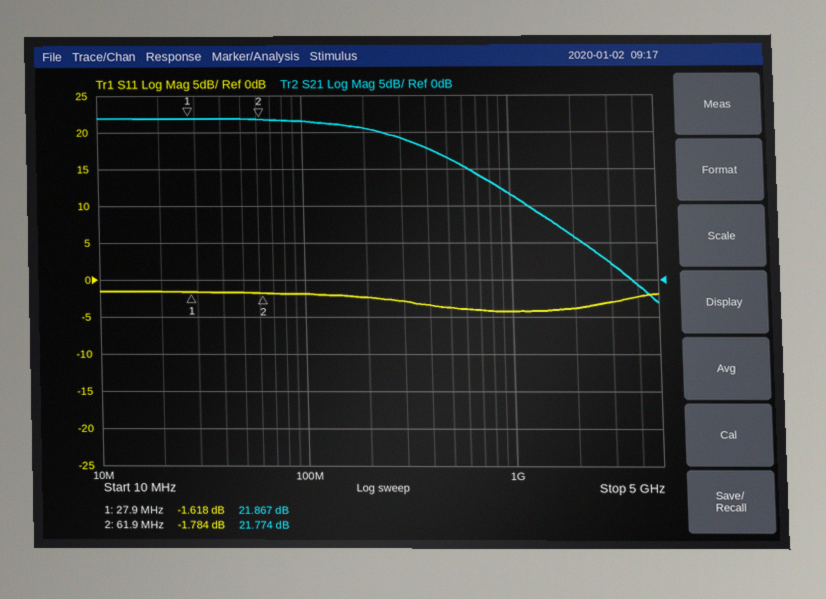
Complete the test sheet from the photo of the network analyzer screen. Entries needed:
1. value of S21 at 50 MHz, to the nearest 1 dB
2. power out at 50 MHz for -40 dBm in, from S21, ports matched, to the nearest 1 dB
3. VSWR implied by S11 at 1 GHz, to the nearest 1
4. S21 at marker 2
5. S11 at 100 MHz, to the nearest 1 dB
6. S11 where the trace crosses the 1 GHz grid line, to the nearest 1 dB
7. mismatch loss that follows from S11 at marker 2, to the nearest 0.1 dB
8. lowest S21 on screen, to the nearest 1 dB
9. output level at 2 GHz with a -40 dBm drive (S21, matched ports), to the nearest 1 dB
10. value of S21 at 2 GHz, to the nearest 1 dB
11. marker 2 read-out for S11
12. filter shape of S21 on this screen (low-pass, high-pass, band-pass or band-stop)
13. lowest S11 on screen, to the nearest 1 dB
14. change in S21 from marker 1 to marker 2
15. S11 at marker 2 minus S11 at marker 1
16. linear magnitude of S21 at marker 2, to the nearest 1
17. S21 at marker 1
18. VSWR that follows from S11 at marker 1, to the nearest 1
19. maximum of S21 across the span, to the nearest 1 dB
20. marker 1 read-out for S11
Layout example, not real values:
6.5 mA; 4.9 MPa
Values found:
22 dB; -18 dBm; 4; 21.774 dB; -2 dB; -4 dB; 4.7 dB; -3 dB; -34 dBm; 6 dB; -1.784 dB; low-pass; -4 dB; -0.093 dB; -0.166 dB; 12; 21.867 dB; 11; 22 dB; -1.618 dB
